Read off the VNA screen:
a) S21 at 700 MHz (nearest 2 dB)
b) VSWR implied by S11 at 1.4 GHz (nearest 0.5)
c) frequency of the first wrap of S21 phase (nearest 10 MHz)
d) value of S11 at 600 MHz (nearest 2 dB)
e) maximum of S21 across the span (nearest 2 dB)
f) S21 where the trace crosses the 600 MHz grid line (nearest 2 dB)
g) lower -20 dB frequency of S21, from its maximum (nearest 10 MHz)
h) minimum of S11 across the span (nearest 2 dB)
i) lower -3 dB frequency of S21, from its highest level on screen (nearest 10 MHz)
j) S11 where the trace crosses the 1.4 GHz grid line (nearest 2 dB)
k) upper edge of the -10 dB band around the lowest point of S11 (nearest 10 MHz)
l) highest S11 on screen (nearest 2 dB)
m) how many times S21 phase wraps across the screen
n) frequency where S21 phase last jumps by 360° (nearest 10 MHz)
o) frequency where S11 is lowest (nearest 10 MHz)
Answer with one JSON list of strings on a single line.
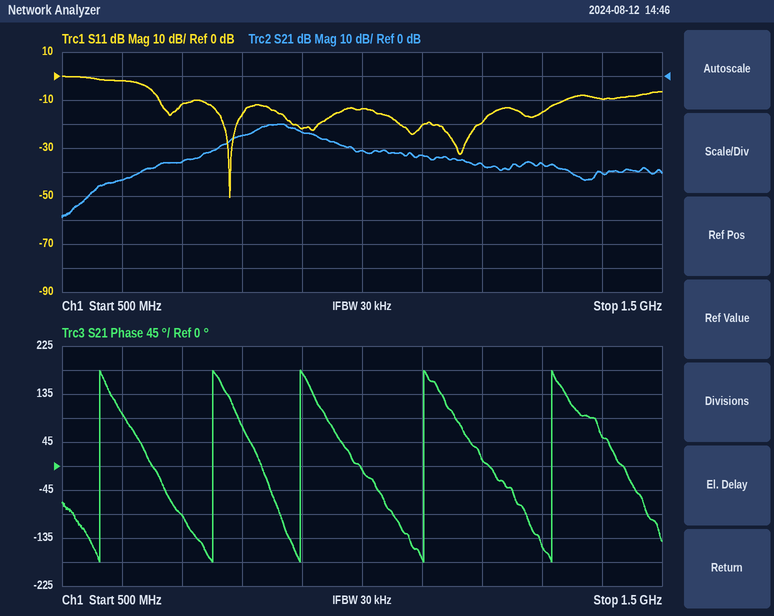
["-36 dB", "2.0", "560 MHz", "-2 dB", "-20 dB", "-44 dB", "630 MHz", "-50 dB", "820 MHz", "-10 dB", "1.34 GHz", "0 dB", "5", "1.32 GHz", "780 MHz"]
